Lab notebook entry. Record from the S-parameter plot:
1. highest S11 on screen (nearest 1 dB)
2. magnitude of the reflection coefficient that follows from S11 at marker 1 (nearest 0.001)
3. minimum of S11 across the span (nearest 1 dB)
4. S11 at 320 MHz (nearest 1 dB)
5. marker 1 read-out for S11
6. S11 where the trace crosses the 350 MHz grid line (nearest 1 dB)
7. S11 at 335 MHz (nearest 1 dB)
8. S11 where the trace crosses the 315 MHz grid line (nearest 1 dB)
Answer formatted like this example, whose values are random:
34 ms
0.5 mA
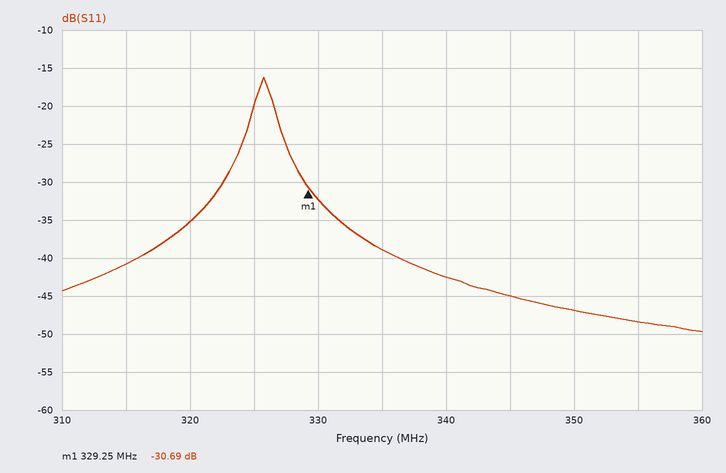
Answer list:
-16 dB
0.029
-50 dB
-35 dB
-30.69 dB
-47 dB
-39 dB
-41 dB
